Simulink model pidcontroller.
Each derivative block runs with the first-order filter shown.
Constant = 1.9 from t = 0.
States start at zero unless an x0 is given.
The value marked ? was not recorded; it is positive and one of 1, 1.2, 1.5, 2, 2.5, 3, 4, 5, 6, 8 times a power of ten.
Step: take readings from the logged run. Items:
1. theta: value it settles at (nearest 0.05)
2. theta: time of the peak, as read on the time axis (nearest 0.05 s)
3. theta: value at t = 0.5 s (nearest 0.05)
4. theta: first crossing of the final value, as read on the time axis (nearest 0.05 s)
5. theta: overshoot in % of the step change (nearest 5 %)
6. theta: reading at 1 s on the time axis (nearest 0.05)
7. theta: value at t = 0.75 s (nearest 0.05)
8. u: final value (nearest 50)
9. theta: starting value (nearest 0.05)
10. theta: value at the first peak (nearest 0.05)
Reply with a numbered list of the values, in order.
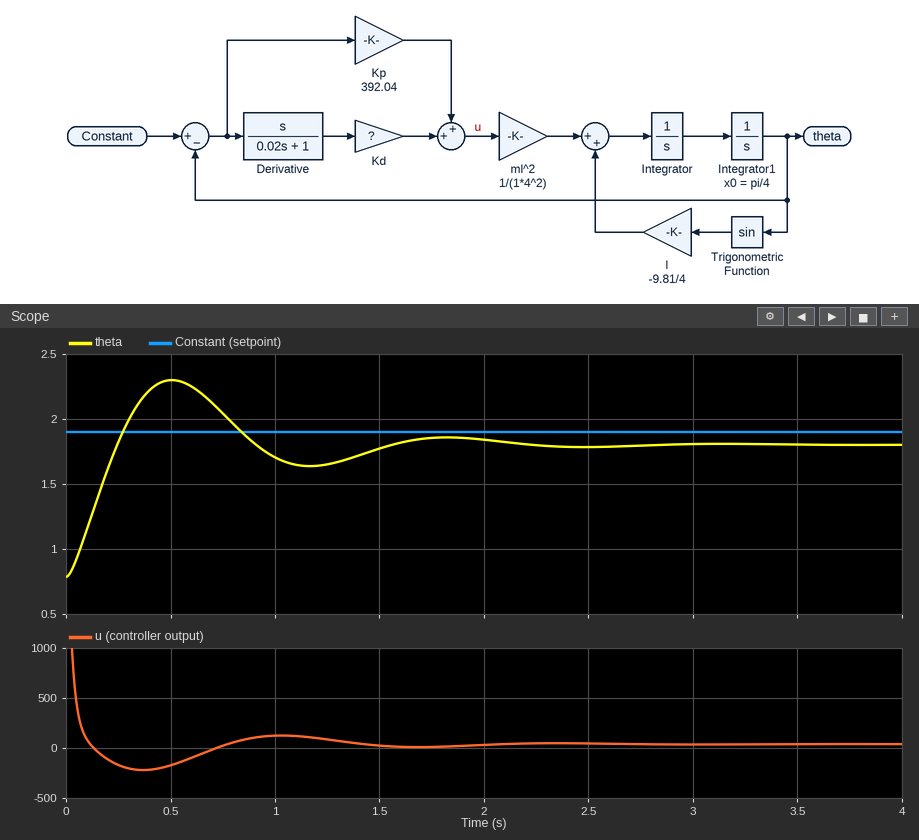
1. 1.80
2. 0.50 s
3. 2.30
4. 0.25 s
5. 50 %
6. 1.70
7. 2.05
8. 50
9. 0.80
10. 2.30
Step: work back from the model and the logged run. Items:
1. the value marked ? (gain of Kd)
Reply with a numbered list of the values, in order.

1. 50
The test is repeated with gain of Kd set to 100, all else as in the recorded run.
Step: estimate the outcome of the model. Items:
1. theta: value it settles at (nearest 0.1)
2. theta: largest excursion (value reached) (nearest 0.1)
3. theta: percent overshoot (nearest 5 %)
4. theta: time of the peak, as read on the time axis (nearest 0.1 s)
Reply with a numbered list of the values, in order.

1. 1.8
2. 2.1
3. 30 %
4. 0.4 s
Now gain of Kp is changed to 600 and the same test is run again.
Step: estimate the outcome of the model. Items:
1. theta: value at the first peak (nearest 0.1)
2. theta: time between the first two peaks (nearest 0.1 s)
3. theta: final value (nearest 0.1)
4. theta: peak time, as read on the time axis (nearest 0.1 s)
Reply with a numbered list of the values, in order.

1. 2.4
2. 1.0 s
3. 1.8
4. 0.4 s
